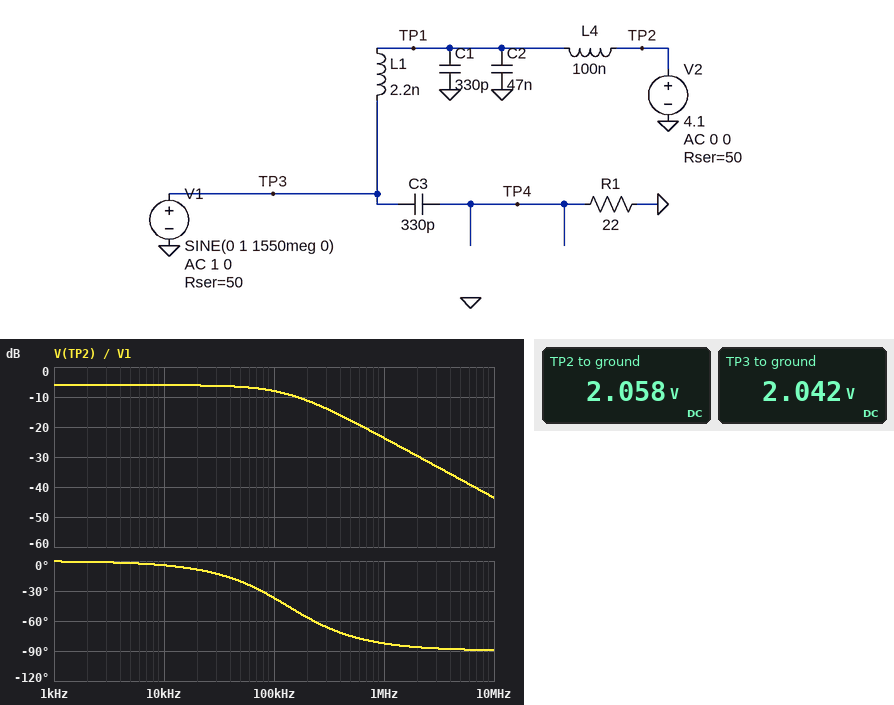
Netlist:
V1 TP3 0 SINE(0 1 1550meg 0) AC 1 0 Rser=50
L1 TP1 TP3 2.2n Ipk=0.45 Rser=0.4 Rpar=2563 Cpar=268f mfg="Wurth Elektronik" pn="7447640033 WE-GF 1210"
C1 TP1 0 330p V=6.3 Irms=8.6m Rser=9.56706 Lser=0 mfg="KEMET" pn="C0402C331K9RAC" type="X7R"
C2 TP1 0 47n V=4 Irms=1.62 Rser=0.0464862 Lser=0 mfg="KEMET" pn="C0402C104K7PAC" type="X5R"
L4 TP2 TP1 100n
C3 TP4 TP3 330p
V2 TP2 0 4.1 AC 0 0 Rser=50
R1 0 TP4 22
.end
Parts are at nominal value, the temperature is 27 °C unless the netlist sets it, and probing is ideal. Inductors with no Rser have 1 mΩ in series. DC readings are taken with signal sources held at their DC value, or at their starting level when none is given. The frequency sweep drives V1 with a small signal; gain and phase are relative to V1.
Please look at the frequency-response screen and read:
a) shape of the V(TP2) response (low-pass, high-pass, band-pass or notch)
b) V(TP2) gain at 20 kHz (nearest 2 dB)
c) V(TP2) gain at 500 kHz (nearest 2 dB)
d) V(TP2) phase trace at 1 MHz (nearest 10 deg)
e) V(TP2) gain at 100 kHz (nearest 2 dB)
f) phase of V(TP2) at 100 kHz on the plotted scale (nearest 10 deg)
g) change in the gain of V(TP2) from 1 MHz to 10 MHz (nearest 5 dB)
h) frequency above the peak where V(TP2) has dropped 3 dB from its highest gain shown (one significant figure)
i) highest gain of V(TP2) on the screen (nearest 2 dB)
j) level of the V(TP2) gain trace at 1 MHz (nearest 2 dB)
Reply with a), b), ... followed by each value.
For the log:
a) low-pass
b) -6 dB
c) -18 dB
d) -80 deg
e) -8 dB
f) -40 deg
g) -20 dB
h) 100 kHz
i) -6 dB
j) -24 dB
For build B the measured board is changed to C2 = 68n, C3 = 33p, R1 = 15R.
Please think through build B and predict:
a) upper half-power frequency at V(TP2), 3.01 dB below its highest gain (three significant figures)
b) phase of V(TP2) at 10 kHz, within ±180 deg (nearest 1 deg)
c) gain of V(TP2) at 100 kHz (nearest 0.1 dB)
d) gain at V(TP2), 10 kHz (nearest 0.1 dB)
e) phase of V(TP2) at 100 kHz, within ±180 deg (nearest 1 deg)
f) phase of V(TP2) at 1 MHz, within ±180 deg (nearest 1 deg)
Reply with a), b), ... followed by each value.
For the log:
a) 92.6 kHz
b) -6 deg
c) -9.4 dB
d) -6.1 dB
e) -47 deg
f) -84 deg
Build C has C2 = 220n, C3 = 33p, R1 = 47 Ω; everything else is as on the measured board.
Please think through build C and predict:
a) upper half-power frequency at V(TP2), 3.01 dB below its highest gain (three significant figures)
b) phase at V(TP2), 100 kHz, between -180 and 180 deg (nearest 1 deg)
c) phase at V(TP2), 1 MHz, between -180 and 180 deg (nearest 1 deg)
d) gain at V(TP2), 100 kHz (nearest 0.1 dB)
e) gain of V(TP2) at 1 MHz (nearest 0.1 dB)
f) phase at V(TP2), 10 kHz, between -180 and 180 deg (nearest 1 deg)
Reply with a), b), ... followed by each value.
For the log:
a) 28.7 kHz
b) -74 deg
c) -85 deg
d) -17.2 dB
e) -36.9 dB
f) -19 deg
